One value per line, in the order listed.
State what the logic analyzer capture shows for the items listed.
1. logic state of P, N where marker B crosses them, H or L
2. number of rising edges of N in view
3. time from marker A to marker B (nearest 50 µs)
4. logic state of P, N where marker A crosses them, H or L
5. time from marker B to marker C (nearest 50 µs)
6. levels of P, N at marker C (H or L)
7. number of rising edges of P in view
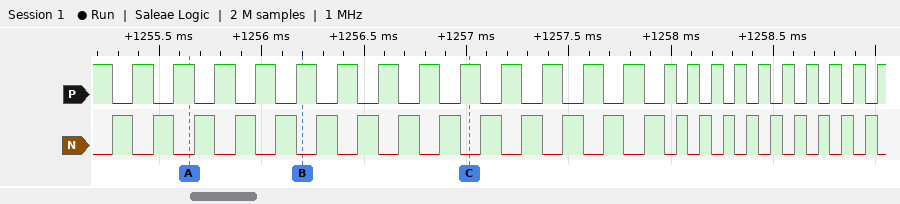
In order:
P=H, N=L
23
550 µs
P=H, N=L
800 µs
P=H, N=L
23
